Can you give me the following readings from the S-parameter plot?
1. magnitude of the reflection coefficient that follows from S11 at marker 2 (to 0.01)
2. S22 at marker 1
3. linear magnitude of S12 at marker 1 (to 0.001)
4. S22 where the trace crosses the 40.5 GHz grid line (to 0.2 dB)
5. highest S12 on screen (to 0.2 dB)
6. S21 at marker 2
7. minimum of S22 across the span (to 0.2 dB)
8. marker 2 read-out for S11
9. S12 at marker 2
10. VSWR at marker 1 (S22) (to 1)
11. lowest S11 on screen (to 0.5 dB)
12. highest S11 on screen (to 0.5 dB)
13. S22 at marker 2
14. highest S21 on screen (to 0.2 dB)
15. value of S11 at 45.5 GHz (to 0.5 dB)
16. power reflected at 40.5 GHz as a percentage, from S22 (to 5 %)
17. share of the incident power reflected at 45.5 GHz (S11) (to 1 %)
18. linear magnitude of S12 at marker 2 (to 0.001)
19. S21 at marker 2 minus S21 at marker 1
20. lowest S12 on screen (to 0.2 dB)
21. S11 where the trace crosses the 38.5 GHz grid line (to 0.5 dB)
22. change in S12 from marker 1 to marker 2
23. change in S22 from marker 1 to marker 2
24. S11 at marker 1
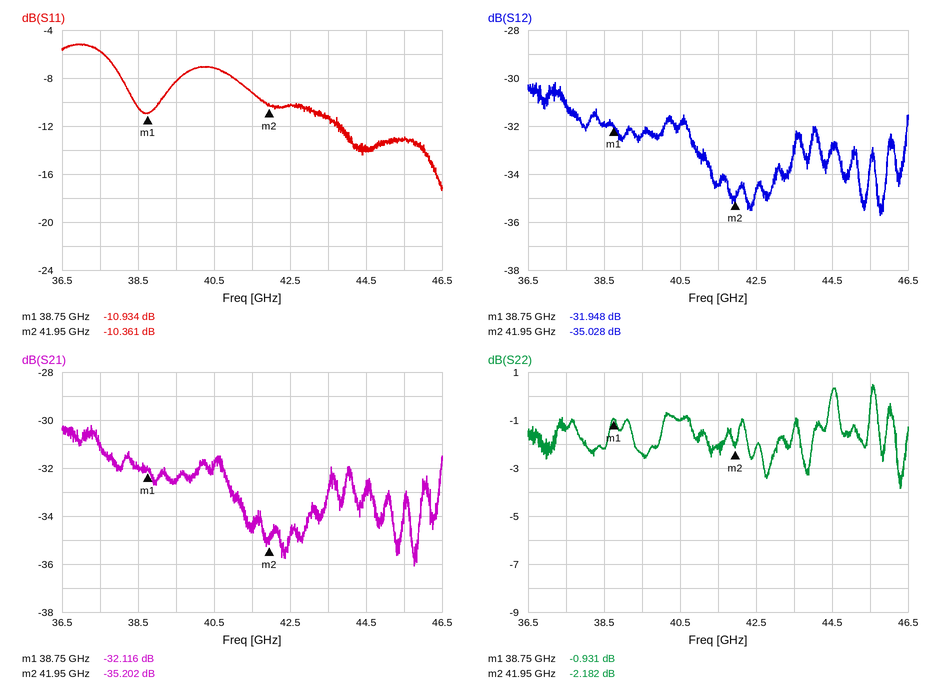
0.30
-0.931 dB
0.025
-1.0 dB
-30.2 dB
-35.202 dB
-3.8 dB
-10.361 dB
-35.028 dB
19
-17.5 dB
-5.0 dB
-2.182 dB
-30.2 dB
-13.0 dB
80 %
5 %
0.018
-3.086 dB
-35.8 dB
-10.5 dB
-3.080 dB
-1.251 dB
-10.934 dB
